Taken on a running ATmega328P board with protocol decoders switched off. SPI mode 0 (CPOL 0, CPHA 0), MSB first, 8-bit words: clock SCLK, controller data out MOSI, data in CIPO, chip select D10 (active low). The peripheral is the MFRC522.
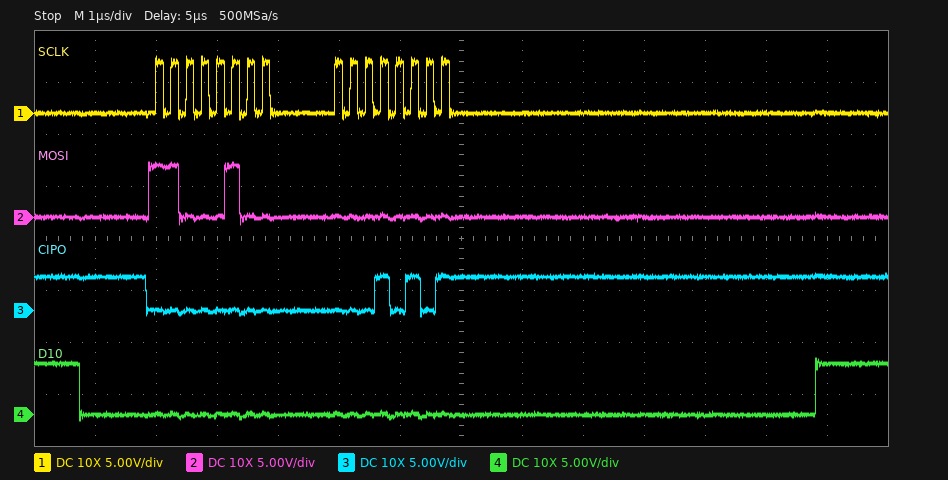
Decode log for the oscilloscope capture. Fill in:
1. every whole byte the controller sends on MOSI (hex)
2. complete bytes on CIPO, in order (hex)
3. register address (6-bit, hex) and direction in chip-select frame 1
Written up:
0xC4 0x00
0x00 0x15
0x22 read
